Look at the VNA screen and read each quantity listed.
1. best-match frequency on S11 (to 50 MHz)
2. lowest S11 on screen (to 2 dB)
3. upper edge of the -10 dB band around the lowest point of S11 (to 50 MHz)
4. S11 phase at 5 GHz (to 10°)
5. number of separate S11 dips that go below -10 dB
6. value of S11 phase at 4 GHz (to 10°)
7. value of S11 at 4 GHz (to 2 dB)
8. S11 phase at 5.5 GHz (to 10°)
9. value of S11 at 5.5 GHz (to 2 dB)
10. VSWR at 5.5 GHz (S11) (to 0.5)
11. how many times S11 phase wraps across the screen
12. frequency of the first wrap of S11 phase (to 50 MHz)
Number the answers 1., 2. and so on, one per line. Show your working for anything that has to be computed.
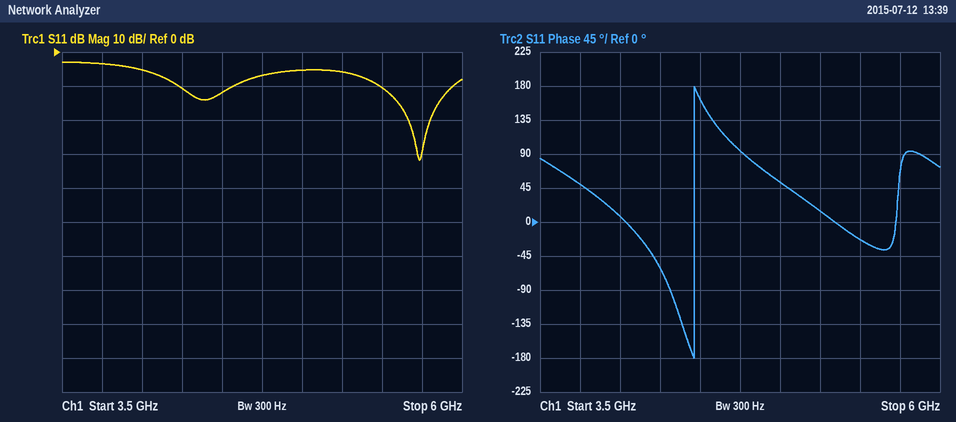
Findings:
1. 5.75 GHz
2. -32 dB
3. 5.95 GHz
4. 50°
5. 2
6. 10°
7. -6 dB
8. -20°
9. -10 dB
10. |Γ| = 10^(-10/20) = 0.3162; VSWR = (1 + 0.3162)/(1 − 0.3162) ≈ 1.92, so 2.0 to the nearest 0.5
11. 1
12. 4.45 GHz
